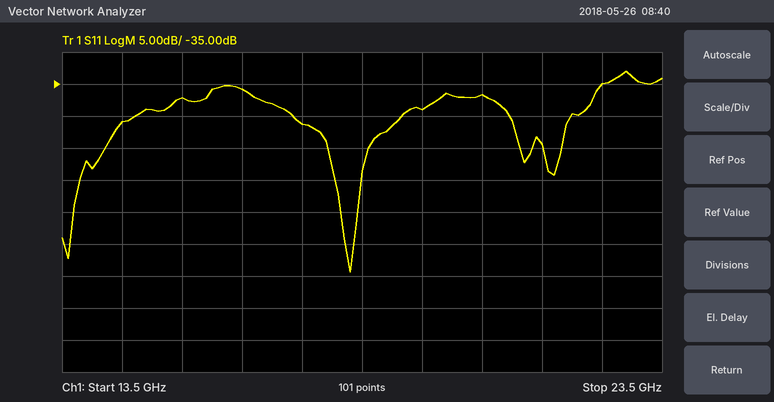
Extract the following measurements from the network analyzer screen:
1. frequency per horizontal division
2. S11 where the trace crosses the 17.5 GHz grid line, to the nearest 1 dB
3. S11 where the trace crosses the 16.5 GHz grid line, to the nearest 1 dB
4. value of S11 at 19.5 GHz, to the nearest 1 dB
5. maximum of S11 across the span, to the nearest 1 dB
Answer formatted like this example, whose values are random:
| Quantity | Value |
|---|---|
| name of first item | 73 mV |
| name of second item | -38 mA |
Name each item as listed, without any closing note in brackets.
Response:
| Quantity | Value |
|---|---|
| frequency per horizontal division | 1 GHz |
| S11 where the trace crosses the 17.5 GHz grid line, to the nearest 1 dB | -41 dB |
| S11 where the trace crosses the 16.5 GHz grid line, to the nearest 1 dB | -36 dB |
| value of S11 at 19.5 GHz, to the nearest 1 dB | -39 dB |
| maximum of S11 across the span, to the nearest 1 dB | -33 dB |
